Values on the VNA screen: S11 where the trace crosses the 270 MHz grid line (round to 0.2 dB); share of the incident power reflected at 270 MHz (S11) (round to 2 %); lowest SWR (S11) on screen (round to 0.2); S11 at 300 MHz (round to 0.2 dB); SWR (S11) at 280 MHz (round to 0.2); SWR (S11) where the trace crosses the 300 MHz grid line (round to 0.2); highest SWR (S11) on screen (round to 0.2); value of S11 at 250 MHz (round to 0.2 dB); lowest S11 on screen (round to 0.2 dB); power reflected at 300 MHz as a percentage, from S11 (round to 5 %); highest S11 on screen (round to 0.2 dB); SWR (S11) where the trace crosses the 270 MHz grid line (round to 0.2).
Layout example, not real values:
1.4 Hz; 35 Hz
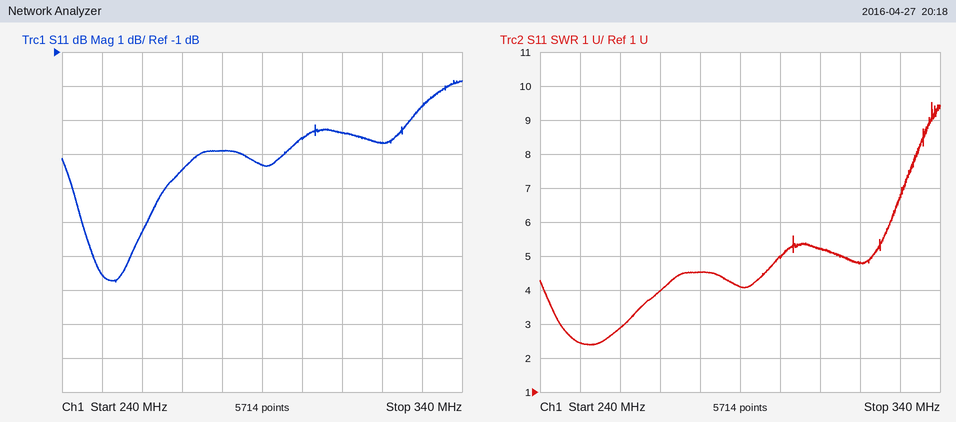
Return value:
-4.4 dB; 36 %; 2.4; -3.6 dB; 4.6; 5.0; 9.6; -7.6 dB; -7.8 dB; 45 %; -1.8 dB; 4.0
